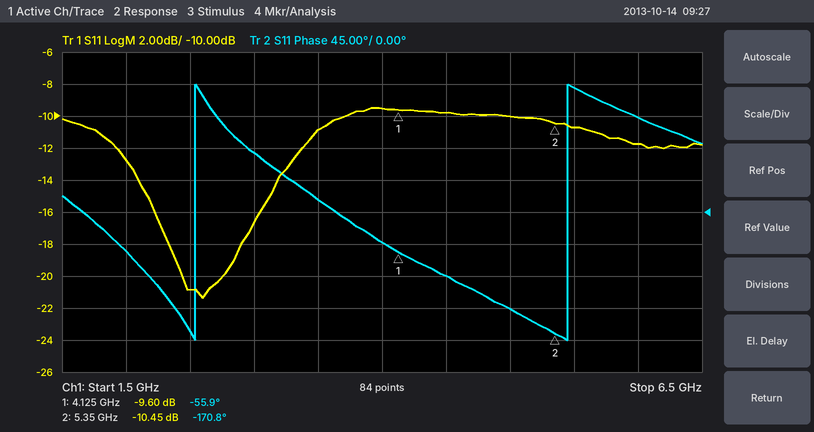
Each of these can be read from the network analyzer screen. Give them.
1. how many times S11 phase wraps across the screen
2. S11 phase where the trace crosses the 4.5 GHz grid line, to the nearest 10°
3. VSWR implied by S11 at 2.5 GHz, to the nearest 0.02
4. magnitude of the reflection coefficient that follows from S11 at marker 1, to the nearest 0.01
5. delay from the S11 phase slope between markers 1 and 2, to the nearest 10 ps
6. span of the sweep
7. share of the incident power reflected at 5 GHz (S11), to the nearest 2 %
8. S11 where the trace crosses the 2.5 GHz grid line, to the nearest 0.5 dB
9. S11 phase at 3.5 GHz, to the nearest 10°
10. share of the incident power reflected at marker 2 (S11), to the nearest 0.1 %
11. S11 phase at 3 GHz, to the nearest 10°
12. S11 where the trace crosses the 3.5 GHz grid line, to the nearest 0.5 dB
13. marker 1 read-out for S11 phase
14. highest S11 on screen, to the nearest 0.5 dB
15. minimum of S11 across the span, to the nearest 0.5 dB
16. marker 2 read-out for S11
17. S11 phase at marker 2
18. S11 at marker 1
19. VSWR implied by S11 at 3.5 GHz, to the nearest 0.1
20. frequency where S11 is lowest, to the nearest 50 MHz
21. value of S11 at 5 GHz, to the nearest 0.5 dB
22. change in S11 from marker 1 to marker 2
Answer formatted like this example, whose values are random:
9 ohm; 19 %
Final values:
2; -90°; 1.20; 0.33; 260 ps; 5 GHz; 10 %; -21.0 dB; 20°; 9.0 %; 80°; -11.0 dB; -55.9°; -9.5 dB; -21.5 dB; -10.45 dB; -170.8°; -9.60 dB; 1.8; 2.60 GHz; -10.0 dB; -0.85 dB
